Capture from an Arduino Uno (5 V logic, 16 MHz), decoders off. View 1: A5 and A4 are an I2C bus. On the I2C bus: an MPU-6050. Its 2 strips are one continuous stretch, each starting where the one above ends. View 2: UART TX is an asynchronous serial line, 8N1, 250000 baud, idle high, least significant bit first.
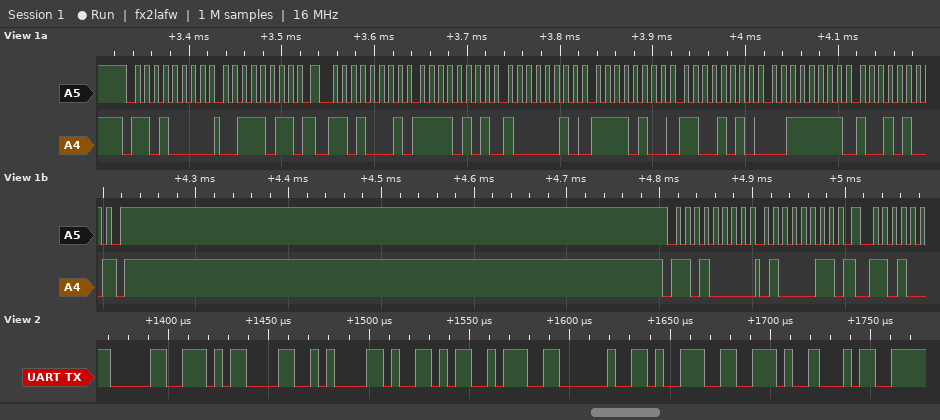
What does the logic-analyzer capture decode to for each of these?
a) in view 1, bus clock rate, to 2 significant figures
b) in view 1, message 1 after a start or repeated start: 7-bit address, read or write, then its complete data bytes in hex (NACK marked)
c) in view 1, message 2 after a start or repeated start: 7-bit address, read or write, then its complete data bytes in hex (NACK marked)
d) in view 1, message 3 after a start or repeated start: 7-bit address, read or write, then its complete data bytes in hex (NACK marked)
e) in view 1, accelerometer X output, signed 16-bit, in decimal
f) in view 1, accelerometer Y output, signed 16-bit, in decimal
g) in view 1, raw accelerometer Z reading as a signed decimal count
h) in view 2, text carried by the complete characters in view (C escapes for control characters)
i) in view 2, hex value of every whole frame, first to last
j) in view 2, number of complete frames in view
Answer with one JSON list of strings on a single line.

["100 kHz", "0x68 write: 3B", "0x68 read: F5 82 F4 CA 3F 94 NACK", "0x68 write: 43", "-2686", "-2870", "16276", "\"0\\r\\nY: 9.4\"", "0x30 0x0D 0x0A 0x59 0x3A 0x20 0x39 0x2E 0x34", "9"]
